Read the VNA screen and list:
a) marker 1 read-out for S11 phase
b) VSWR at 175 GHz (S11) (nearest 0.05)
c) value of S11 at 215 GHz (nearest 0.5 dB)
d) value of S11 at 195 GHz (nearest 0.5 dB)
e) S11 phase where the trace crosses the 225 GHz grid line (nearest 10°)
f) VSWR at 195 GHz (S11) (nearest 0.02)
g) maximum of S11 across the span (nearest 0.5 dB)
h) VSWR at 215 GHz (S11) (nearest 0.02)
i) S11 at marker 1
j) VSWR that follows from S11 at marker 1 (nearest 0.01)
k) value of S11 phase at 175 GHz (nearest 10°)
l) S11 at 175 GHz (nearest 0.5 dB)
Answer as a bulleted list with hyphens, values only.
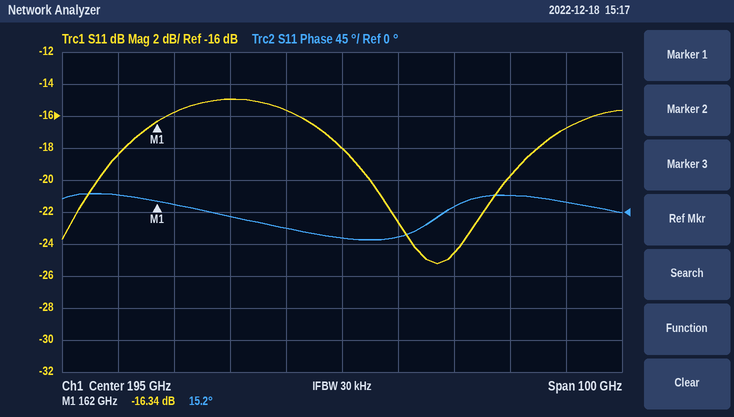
- 15.2°
- 1.45
- -24.5 dB
- -18.0 dB
- 20°
- 1.28
- -15.0 dB
- 1.12
- -16.34 dB
- 1.36
- -10°
- -15.0 dB
